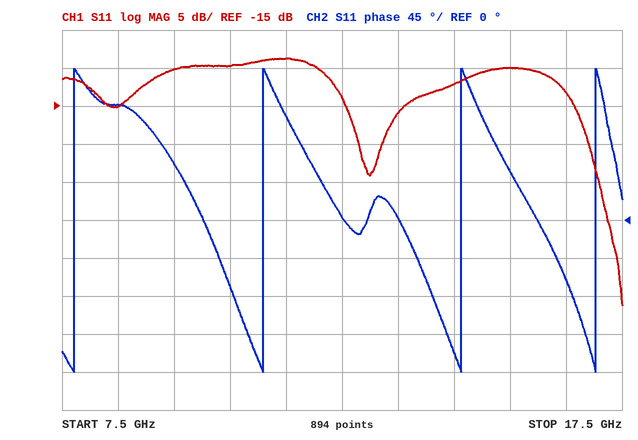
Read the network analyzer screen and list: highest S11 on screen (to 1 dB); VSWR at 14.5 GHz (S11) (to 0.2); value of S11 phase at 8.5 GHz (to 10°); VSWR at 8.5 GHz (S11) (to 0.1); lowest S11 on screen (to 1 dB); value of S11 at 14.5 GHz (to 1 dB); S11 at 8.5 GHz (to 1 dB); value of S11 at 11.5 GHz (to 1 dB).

-9 dB
1.6
140°
1.4
-41 dB
-12 dB
-15 dB
-9 dB
